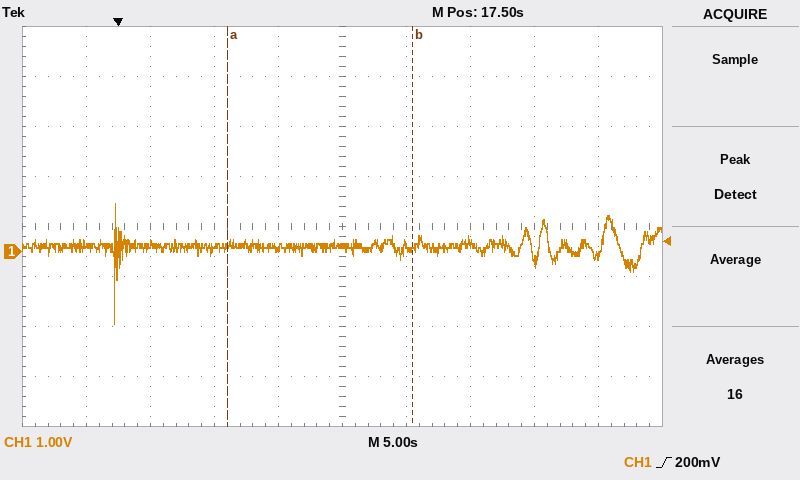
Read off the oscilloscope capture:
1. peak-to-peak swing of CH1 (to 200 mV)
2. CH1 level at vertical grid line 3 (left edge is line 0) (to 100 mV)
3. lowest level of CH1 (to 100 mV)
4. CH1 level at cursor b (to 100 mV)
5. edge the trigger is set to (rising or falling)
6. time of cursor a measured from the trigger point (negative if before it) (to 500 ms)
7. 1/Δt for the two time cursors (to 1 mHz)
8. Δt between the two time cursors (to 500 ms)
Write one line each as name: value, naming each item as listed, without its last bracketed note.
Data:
peak-to-peak swing of CH1: 2.4 V
CH1 level at vertical grid line 3 (left edge is line 0): 100 mV
lowest level of CH1: -1.4 V
CH1 level at cursor b: 100 mV
edge the trigger is set to: rising
time of cursor a measured from the trigger point (negative if before it): +8.5 s
1/Δt for the two time cursors: 69 mHz
Δt between the two time cursors: 14.5 s
